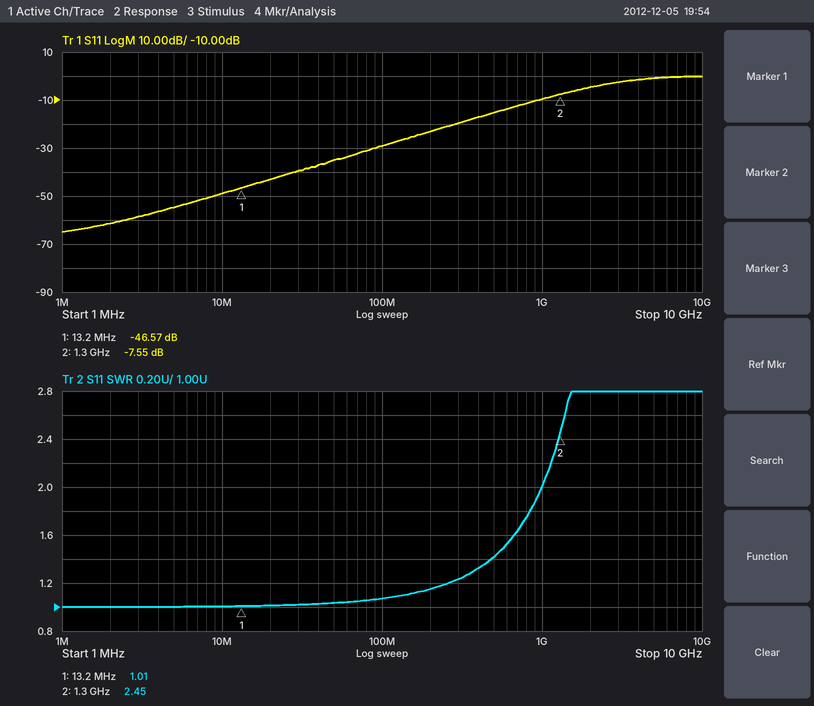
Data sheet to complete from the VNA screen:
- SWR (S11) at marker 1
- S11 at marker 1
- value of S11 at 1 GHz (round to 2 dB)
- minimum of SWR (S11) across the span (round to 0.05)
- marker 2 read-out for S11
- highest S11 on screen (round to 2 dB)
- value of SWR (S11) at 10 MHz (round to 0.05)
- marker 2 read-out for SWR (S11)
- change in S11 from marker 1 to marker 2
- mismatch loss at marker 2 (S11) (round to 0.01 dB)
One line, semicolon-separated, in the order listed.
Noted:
1.01; -46.57 dB; -10 dB; 1.00; -7.55 dB; 0 dB; 1.00; 2.45; 39.02 dB; 0.84 dB
